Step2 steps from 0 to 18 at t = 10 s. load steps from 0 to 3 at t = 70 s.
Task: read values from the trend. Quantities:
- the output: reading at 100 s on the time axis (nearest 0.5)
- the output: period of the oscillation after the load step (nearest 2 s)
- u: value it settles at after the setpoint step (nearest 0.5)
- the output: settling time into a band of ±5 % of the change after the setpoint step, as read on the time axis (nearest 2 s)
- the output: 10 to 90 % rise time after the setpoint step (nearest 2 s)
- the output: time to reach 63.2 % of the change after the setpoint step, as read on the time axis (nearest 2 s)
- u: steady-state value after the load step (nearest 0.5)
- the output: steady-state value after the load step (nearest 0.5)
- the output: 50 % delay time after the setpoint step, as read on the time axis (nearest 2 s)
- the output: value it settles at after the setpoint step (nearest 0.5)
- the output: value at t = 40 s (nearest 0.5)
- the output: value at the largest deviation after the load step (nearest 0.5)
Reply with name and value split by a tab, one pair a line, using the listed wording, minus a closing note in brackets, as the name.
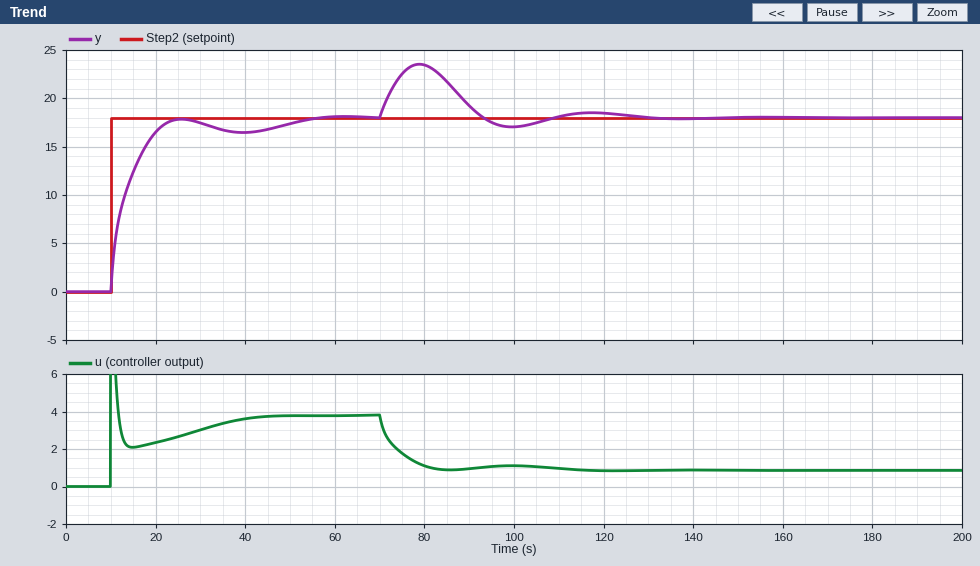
the output: reading at 100 s on the time axis	17.0
the output: period of the oscillation after the load step	38 s
u: value it settles at after the setpoint step	4.0
the output: settling time into a band of ±5 % of the change after the setpoint step, as read on the time axis	48 s
the output: 10 to 90 % rise time after the setpoint step	10 s
the output: time to reach 63.2 % of the change after the setpoint step, as read on the time axis	14 s
u: steady-state value after the load step	1.0
the output: steady-state value after the load step	18.0
the output: 50 % delay time after the setpoint step, as read on the time axis	12 s
the output: value it settles at after the setpoint step	18.0
the output: value at t = 40 s	16.5
the output: value at the largest deviation after the load step	23.5
